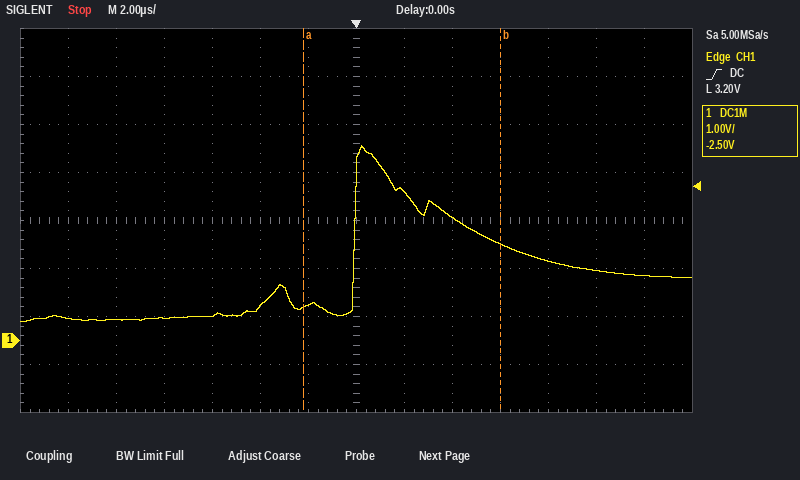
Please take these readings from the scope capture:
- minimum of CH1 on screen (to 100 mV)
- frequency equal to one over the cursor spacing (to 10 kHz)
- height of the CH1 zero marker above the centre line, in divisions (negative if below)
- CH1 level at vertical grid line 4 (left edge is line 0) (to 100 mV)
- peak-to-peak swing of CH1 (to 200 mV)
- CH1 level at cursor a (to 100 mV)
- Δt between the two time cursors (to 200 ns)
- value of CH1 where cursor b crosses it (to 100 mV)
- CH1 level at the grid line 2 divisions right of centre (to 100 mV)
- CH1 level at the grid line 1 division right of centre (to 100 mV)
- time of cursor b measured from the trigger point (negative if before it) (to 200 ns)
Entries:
400 mV
120 kHz
-2.5 div
500 mV
3.6 V
700 mV
8.2 µs
2.0 V
2.6 V
3.1 V
+6.0 µs
